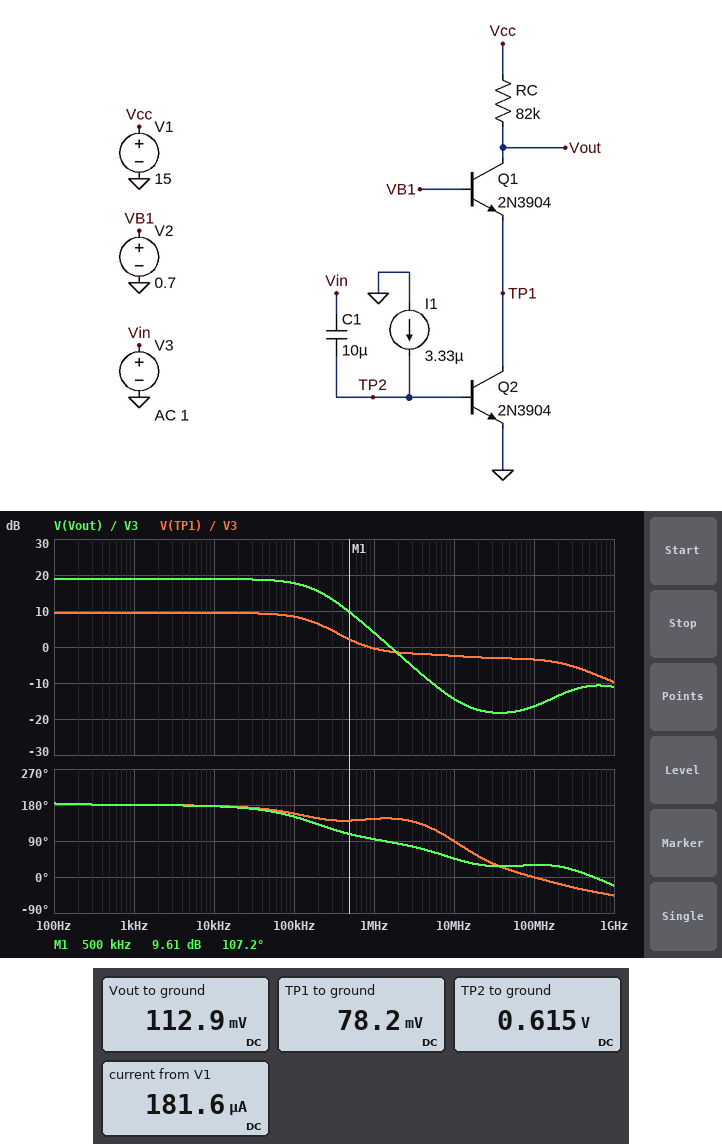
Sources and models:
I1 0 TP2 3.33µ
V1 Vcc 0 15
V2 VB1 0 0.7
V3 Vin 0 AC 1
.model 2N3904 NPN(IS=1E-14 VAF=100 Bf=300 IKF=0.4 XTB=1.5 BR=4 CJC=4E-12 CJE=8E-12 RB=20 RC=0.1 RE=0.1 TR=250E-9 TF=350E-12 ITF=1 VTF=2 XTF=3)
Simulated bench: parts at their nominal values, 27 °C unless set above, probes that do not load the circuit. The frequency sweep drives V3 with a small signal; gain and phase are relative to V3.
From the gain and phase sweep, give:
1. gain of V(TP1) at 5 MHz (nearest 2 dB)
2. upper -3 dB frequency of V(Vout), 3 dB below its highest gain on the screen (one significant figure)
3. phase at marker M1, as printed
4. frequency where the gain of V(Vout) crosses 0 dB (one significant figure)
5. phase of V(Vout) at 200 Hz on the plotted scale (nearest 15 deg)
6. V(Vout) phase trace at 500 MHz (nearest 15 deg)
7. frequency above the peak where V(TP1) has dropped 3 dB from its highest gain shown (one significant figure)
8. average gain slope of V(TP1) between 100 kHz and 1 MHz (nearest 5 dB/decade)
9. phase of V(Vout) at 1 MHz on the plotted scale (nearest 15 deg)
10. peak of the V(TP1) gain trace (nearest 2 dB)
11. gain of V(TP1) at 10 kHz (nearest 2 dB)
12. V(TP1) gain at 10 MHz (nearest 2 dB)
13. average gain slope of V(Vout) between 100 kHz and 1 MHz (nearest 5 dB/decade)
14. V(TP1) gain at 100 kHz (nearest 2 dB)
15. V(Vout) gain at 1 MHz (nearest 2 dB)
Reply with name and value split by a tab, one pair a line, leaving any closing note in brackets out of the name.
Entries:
gain of V(TP1) at 5 MHz	-2 dB
upper -3 dB frequency of V(Vout), 3 dB below its highest gain on the screen	200 kHz
phase at marker M1, as printed	107.2 deg
frequency where the gain of V(Vout) crosses 0 dB	2 MHz
phase of V(Vout) at 200 Hz on the plotted scale	180 deg
V(Vout) phase trace at 500 MHz	0 deg
frequency above the peak where V(TP1) has dropped 3 dB from its highest gain shown	200 kHz
average gain slope of V(TP1) between 100 kHz and 1 MHz	-10 dB/decade
phase of V(Vout) at 1 MHz on the plotted scale	90 deg
peak of the V(TP1) gain trace	10 dB
gain of V(TP1) at 10 kHz	10 dB
V(TP1) gain at 10 MHz	-2 dB
average gain slope of V(Vout) between 100 kHz and 1 MHz	-15 dB/decade
V(TP1) gain at 100 kHz	8 dB
V(Vout) gain at 1 MHz	4 dB
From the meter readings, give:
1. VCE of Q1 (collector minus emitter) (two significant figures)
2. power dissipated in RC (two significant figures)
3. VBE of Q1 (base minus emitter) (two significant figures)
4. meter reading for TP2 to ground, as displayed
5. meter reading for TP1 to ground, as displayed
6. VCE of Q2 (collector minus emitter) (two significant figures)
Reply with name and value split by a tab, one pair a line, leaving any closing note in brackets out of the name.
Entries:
VCE of Q1 (collector minus emitter)	35 mV
power dissipated in RC	2.7 mW
VBE of Q1 (base minus emitter)	620 mV
meter reading for TP2 to ground, as displayed	0.615 V
meter reading for TP1 to ground, as displayed	78.2 mV
VCE of Q2 (collector minus emitter)	78 mV
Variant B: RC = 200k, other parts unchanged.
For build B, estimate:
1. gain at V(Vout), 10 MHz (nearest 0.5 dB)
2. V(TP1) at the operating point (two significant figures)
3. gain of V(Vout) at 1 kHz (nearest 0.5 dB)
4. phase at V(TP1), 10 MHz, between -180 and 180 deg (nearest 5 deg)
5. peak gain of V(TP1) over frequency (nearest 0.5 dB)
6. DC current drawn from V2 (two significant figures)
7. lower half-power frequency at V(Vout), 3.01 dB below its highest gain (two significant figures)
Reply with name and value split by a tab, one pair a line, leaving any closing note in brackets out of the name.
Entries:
gain at V(Vout), 10 MHz	-17.5 dB
V(TP1) at the operating point	68 mV
gain of V(Vout) at 1 kHz	5.5 dB
phase at V(TP1), 10 MHz, between -180 and 180 deg	85 deg
peak gain of V(TP1) over frequency	4.0 dB
DC current drawn from V2	65 µA
lower half-power frequency at V(Vout), 3.01 dB below its highest gain	4.7 Hz
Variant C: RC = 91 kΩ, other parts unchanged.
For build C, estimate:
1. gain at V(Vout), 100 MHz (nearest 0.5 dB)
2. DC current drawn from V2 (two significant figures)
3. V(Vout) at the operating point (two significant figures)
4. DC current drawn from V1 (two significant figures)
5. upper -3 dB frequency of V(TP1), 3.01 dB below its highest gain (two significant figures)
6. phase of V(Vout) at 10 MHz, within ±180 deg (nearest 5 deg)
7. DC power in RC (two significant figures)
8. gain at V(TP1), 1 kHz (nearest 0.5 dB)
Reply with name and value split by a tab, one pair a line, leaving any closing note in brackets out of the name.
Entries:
gain at V(Vout), 100 MHz	-16.0 dB
DC current drawn from V2	26 µA
V(Vout) at the operating point	100 mV
DC current drawn from V1	160 µA
upper -3 dB frequency of V(TP1), 3.01 dB below its highest gain	200 kHz
phase of V(Vout) at 10 MHz, within ±180 deg	55 deg
DC power in RC	2.4 mW
gain at V(TP1), 1 kHz	8.5 dB
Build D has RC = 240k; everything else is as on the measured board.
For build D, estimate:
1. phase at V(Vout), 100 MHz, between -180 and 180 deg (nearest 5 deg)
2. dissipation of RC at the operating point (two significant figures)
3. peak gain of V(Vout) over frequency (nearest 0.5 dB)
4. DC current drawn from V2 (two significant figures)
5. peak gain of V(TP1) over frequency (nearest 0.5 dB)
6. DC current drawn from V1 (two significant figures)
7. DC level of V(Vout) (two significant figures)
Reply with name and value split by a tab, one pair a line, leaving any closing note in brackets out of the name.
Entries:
phase at V(Vout), 100 MHz, between -180 and 180 deg	25 deg
dissipation of RC at the operating point	930 µW
peak gain of V(Vout) over frequency	4.5 dB
DC current drawn from V2	71 µA
peak gain of V(TP1) over frequency	3.0 dB
DC current drawn from V1	62 µA
DC level of V(Vout)	77 mV
